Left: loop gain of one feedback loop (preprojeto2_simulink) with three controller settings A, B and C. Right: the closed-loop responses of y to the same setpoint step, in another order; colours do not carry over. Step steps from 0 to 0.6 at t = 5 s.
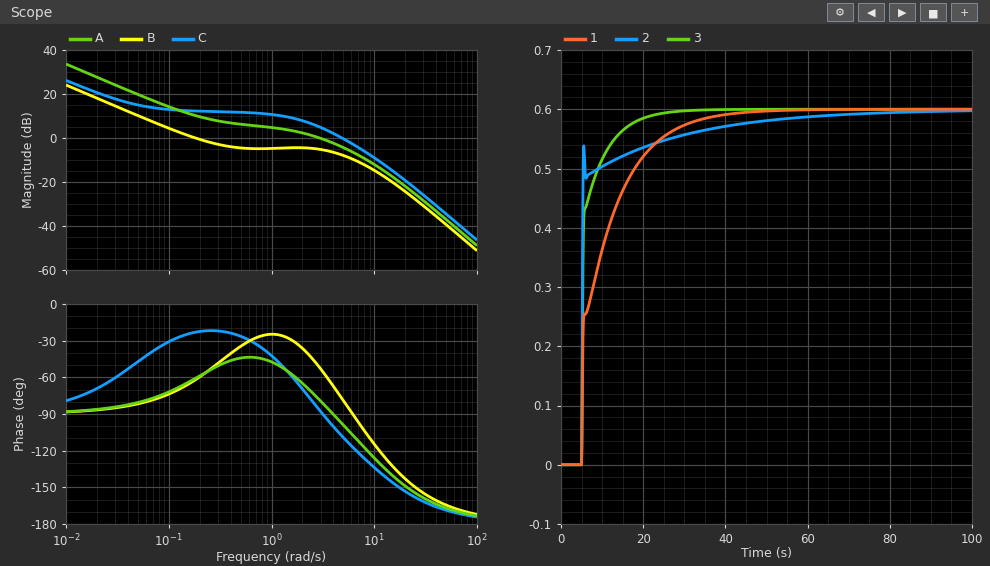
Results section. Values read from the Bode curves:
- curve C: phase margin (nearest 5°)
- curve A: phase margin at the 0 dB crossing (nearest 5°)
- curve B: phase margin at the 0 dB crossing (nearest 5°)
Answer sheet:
70°
100°
120°
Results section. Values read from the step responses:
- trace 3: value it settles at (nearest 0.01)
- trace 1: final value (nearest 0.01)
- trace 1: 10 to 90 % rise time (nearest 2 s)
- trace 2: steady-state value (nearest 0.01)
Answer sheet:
0.60
0.60
18 s
0.60
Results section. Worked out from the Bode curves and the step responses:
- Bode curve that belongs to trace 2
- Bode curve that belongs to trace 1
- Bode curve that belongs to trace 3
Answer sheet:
C
B
A
